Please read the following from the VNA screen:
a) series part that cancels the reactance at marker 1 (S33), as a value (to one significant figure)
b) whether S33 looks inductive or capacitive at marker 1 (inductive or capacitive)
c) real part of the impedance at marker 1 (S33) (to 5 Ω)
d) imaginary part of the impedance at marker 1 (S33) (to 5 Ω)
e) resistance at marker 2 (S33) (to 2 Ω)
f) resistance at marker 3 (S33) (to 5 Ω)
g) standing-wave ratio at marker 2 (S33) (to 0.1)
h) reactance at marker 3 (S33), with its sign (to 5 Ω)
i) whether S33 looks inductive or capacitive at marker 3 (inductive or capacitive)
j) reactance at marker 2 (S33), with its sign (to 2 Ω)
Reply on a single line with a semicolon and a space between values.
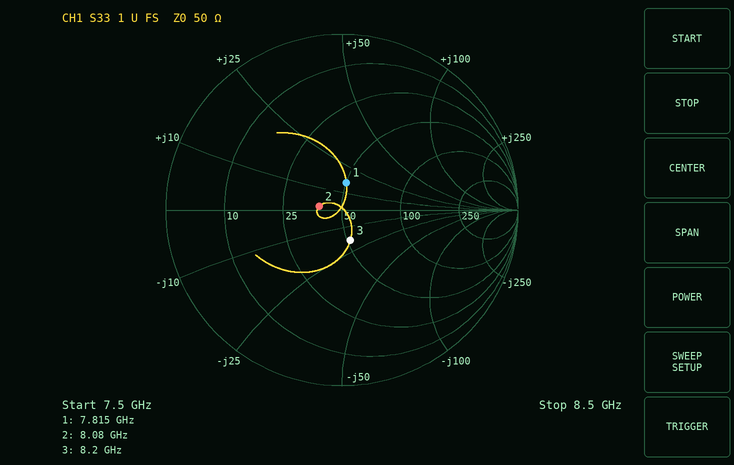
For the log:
1 pF; inductive; 50 Ω; +15 Ω; 38 Ω; 50 Ω; 1.3; -20 Ω; capacitive; +2 Ω
